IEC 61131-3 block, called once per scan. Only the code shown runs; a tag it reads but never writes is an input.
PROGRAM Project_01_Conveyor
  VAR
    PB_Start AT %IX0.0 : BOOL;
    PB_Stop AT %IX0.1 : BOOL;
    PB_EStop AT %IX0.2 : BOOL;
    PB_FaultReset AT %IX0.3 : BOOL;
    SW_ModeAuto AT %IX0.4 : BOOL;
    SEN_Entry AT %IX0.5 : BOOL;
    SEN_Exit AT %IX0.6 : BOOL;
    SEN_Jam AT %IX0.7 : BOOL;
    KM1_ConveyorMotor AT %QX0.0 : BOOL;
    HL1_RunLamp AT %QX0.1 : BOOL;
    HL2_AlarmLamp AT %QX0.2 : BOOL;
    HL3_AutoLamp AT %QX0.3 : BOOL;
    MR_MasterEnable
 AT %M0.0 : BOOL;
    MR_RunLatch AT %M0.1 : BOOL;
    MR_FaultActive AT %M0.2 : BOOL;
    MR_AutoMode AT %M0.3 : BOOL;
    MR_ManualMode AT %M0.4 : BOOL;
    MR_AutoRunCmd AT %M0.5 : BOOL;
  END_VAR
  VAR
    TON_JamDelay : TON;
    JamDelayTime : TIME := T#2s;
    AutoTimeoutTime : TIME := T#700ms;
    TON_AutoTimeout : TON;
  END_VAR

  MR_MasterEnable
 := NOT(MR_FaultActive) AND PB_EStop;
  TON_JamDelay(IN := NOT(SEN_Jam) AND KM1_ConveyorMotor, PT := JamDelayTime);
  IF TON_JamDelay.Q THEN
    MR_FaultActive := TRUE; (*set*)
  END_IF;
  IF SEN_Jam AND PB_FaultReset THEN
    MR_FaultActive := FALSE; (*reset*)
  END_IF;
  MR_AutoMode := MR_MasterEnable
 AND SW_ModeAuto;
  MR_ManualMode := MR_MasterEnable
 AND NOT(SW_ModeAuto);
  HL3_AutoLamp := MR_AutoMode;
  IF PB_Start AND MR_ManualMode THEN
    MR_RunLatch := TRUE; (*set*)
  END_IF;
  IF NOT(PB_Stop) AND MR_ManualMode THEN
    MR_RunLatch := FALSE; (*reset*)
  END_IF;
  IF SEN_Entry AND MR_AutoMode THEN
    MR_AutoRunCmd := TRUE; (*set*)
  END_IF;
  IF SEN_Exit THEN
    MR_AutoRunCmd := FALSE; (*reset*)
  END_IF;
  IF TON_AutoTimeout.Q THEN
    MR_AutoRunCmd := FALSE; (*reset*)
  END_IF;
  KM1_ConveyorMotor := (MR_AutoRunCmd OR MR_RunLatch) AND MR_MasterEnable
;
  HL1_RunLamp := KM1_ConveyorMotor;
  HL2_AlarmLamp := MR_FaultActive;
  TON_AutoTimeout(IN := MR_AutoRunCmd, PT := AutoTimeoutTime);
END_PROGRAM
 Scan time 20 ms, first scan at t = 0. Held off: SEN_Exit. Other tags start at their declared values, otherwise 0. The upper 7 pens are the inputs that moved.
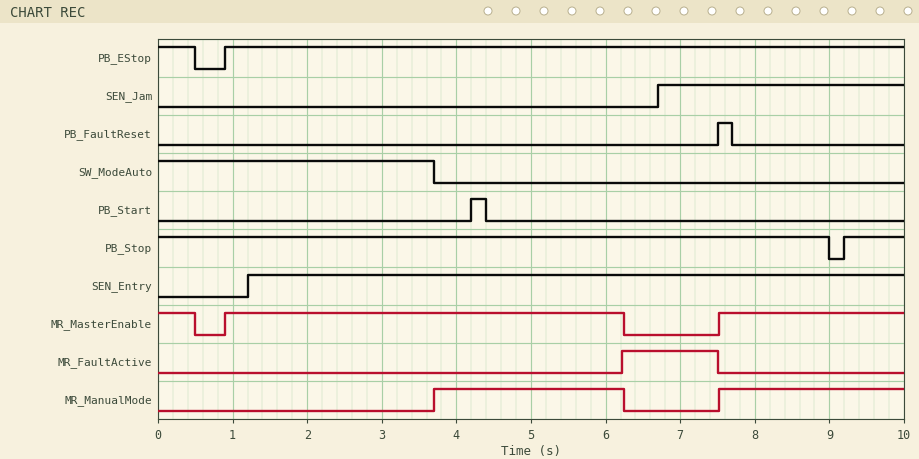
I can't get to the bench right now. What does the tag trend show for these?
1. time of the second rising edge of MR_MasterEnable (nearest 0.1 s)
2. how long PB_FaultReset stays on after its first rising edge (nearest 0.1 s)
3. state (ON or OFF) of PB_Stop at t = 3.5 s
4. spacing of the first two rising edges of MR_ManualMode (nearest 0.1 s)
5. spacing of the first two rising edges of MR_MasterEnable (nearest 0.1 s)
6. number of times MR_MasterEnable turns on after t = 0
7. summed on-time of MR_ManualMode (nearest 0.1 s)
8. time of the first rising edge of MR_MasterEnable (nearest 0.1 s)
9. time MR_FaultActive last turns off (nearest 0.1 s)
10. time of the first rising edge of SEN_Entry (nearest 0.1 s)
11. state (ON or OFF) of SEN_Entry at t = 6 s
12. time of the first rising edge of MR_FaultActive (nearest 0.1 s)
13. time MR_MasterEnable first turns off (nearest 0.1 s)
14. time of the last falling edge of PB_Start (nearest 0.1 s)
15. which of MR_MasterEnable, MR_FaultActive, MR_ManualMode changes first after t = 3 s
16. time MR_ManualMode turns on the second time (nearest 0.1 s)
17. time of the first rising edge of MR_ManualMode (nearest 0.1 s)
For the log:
7.5 s
0.2 s
ON
3.8 s
6.6 s
2
5.0 s
0.9 s
7.5 s
1.2 s
ON
6.2 s
0.5 s
4.4 s
MR_ManualMode
7.5 s
3.7 s
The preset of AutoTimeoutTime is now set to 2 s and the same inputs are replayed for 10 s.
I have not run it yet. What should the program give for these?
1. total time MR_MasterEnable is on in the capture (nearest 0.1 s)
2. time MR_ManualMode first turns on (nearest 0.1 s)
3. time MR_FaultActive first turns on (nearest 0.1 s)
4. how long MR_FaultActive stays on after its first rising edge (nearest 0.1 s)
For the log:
5.3 s
7.5 s
3.2 s
4.3 s
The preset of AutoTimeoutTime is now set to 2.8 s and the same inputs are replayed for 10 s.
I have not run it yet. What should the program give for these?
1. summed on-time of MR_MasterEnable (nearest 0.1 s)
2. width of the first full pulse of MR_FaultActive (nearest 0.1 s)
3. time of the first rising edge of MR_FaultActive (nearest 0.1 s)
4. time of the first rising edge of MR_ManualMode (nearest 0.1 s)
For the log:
5.3 s
4.3 s
3.2 s
7.5 s
